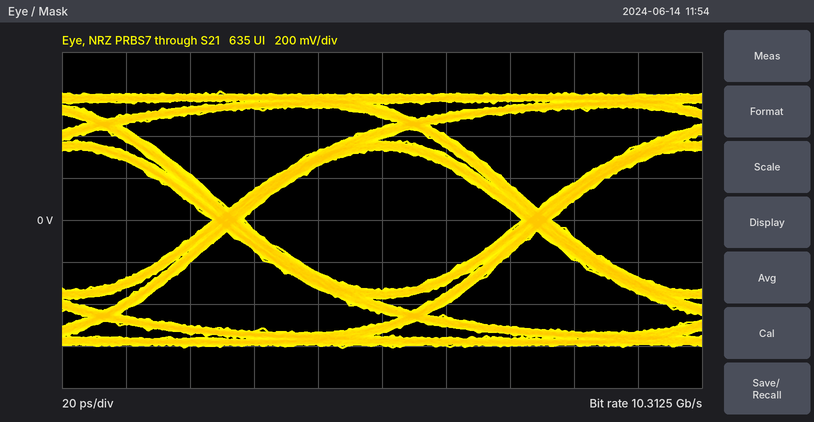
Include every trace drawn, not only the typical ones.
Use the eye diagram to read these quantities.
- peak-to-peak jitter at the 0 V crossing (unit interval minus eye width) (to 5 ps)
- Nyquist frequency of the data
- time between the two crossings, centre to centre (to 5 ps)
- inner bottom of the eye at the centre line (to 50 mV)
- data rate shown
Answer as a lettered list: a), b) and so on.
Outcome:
a) 10 ps
b) 5.15625 GHz
c) 95 ps
d) -350 mV
e) 10.3125 Gb/s
